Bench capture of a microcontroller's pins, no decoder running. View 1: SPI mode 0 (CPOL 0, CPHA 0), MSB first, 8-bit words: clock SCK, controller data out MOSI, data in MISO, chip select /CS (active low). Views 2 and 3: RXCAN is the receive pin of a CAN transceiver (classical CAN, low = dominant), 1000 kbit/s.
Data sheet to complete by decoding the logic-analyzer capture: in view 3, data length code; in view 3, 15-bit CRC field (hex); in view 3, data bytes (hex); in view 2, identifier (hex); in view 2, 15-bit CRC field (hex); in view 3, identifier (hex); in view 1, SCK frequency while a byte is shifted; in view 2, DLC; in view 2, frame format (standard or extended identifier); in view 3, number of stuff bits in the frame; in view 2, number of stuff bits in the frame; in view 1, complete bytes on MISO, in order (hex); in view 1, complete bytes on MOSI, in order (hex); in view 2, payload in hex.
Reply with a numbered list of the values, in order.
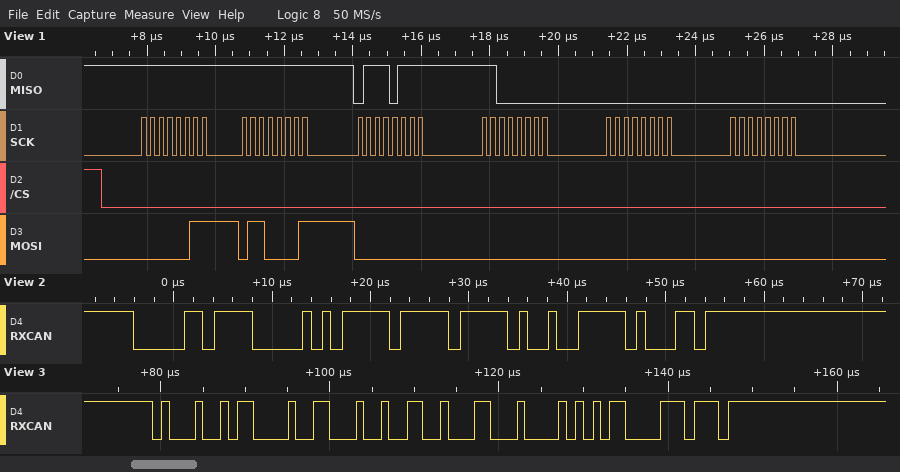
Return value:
1. 4
2. 0x2C3B
3. C4 99 18 85
4. 0x05E
5. 0x13F1
6. 0x44B
7. 4 MHz
8. 2
9. standard
10. 0
11. 6
12. FF FF 77 C0 00 00
13. 03 61 00 00 00 00
14. FF FF
